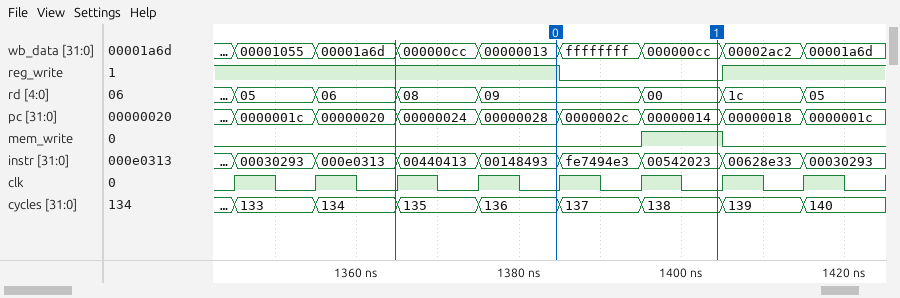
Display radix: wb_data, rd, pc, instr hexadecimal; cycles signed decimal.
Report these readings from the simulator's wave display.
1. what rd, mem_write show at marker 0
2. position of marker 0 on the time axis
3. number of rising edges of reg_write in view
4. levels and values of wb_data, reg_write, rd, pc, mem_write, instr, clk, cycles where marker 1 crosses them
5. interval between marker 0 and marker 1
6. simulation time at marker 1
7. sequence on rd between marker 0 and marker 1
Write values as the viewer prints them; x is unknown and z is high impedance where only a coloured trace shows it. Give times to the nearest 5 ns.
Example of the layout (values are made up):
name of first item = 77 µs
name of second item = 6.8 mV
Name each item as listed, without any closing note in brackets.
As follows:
what rd, mem_write show at marker 0 = rd=09, mem_write=0
position of marker 0 on the time axis = 1385 ns
number of rising edges of reg_write in view = 1
levels and values of wb_data, reg_write, rd, pc, mem_write, instr, clk, cycles where marker 1 crosses them = wb_data=000000cc, reg_write=0, rd=00, pc=00000014, mem_write=1, instr=00542023, clk=0, cycles=138
interval between marker 0 and marker 1 = 20 ns
simulation time at marker 1 = 1405 ns
sequence on rd between marker 0 and marker 1 = 09, 00
